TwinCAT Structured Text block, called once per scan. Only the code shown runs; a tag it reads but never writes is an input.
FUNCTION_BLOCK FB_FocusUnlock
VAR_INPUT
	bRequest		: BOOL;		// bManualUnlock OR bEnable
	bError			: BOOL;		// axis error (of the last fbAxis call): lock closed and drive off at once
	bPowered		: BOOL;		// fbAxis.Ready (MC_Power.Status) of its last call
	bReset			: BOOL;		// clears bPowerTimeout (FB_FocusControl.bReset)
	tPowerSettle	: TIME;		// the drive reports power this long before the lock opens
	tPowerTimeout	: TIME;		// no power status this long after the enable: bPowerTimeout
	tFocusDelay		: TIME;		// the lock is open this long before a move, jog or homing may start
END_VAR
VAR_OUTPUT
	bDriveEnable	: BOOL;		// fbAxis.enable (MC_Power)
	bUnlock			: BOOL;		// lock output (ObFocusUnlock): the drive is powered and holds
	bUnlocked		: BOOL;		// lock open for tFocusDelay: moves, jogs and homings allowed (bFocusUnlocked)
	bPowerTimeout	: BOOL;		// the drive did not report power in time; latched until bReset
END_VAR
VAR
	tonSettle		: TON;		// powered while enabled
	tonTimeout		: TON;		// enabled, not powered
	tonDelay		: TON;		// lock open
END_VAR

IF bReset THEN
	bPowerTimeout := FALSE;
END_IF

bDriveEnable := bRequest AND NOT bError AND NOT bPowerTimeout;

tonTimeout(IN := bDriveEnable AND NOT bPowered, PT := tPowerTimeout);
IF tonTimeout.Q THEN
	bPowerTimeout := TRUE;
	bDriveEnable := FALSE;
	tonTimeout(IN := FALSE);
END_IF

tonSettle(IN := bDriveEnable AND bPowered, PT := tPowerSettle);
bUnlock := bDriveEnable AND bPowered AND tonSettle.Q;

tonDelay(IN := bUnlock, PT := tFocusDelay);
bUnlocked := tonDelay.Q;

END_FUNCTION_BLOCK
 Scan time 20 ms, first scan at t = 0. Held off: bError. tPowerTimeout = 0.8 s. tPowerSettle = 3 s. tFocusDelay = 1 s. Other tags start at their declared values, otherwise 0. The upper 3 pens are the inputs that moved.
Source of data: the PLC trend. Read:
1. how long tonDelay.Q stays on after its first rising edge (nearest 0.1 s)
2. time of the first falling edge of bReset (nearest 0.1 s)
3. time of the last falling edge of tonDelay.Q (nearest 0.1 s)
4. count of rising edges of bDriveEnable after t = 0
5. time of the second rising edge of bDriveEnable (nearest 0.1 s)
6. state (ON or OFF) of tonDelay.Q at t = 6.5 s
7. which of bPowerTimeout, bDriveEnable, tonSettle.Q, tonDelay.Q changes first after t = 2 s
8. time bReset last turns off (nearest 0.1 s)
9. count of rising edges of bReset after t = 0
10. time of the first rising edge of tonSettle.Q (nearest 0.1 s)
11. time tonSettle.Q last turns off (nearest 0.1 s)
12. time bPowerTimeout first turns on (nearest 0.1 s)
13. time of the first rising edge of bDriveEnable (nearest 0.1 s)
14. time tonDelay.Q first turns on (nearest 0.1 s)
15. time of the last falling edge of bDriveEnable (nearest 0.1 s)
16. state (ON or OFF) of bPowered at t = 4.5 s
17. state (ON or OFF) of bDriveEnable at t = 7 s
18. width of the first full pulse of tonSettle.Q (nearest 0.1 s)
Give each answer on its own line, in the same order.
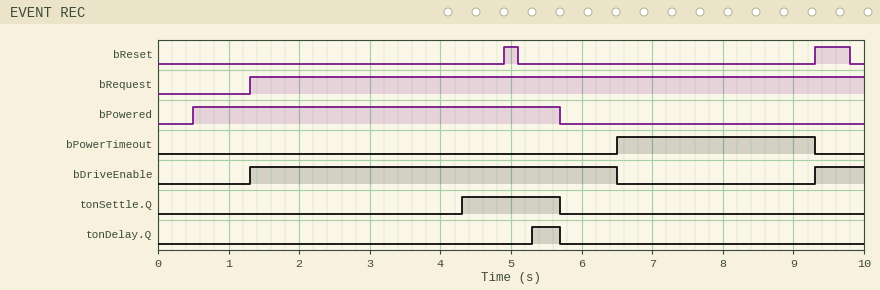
0.4 s
5.1 s
5.7 s
2
9.3 s
OFF
tonSettle.Q
9.8 s
2
4.3 s
5.7 s
6.5 s
1.3 s
5.3 s
6.5 s
ON
OFF
1.4 s
